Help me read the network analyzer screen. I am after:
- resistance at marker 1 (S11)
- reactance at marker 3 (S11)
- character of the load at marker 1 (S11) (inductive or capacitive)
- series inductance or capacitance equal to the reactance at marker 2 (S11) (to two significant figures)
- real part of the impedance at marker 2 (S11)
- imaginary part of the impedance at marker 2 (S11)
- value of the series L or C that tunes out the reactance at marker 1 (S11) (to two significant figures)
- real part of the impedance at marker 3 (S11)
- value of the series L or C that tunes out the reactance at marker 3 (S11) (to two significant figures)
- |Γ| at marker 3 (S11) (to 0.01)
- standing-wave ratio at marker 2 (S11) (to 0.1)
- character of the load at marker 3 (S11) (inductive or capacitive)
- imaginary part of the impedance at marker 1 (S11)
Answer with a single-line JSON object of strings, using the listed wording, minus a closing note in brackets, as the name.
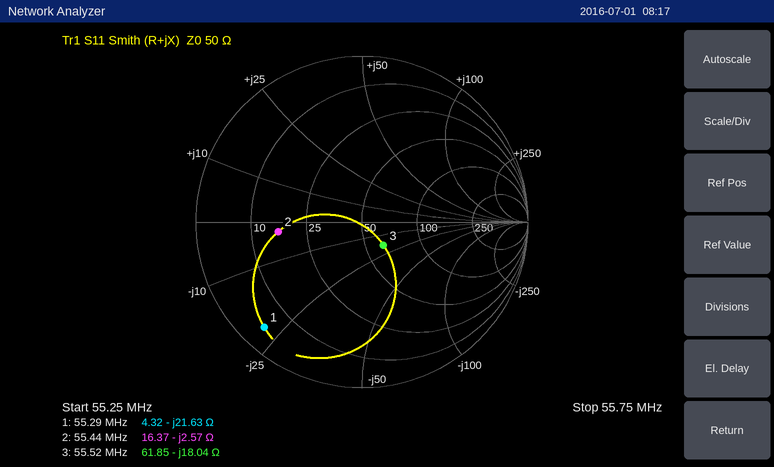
{"resistance at marker 1": "4.32 Ω", "reactance at marker 3": "-18.04 Ω", "character of the load at marker 1 (S11)": "capacitive", "series inductance or capacitance equal to the reactance at marker 2 (S11)": "1.1 nF", "real part of the impedance at marker 2": "16.37 Ω", "imaginary part of the impedance at marker 2": "-2.57 Ω", "value of the series L or C that tunes out the reactance at marker 1 (S11)": "62 nH", "real part of the impedance at marker 3": "61.85 Ω", "value of the series L or C that tunes out the reactance at marker 3 (S11)": "52 nH", "|Γ| at marker 3 (S11)": "0.19", "standing-wave ratio at marker 2 (S11)": "3.1", "character of the load at marker 3 (S11)": "capacitive", "imaginary part of the impedance at marker 1": "-21.63 Ω"}
